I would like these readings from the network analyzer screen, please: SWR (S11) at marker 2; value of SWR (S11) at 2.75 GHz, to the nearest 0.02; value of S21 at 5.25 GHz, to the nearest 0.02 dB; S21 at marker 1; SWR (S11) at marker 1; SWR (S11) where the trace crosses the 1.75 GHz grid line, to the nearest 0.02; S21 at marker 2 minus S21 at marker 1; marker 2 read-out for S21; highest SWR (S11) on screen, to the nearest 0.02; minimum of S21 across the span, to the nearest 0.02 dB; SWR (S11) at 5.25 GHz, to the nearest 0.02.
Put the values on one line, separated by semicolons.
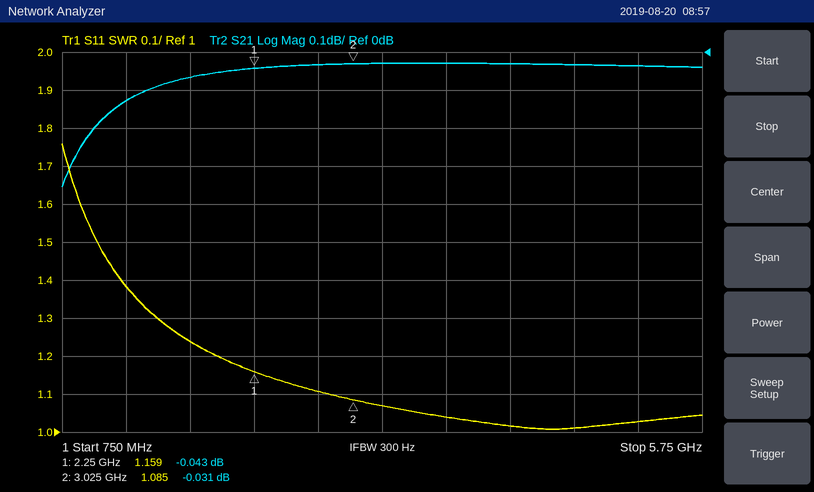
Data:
1.085; 1.10; -0.04 dB; -0.043 dB; 1.159; 1.24; 0.012 dB; -0.031 dB; 1.76; -0.36 dB; 1.02
